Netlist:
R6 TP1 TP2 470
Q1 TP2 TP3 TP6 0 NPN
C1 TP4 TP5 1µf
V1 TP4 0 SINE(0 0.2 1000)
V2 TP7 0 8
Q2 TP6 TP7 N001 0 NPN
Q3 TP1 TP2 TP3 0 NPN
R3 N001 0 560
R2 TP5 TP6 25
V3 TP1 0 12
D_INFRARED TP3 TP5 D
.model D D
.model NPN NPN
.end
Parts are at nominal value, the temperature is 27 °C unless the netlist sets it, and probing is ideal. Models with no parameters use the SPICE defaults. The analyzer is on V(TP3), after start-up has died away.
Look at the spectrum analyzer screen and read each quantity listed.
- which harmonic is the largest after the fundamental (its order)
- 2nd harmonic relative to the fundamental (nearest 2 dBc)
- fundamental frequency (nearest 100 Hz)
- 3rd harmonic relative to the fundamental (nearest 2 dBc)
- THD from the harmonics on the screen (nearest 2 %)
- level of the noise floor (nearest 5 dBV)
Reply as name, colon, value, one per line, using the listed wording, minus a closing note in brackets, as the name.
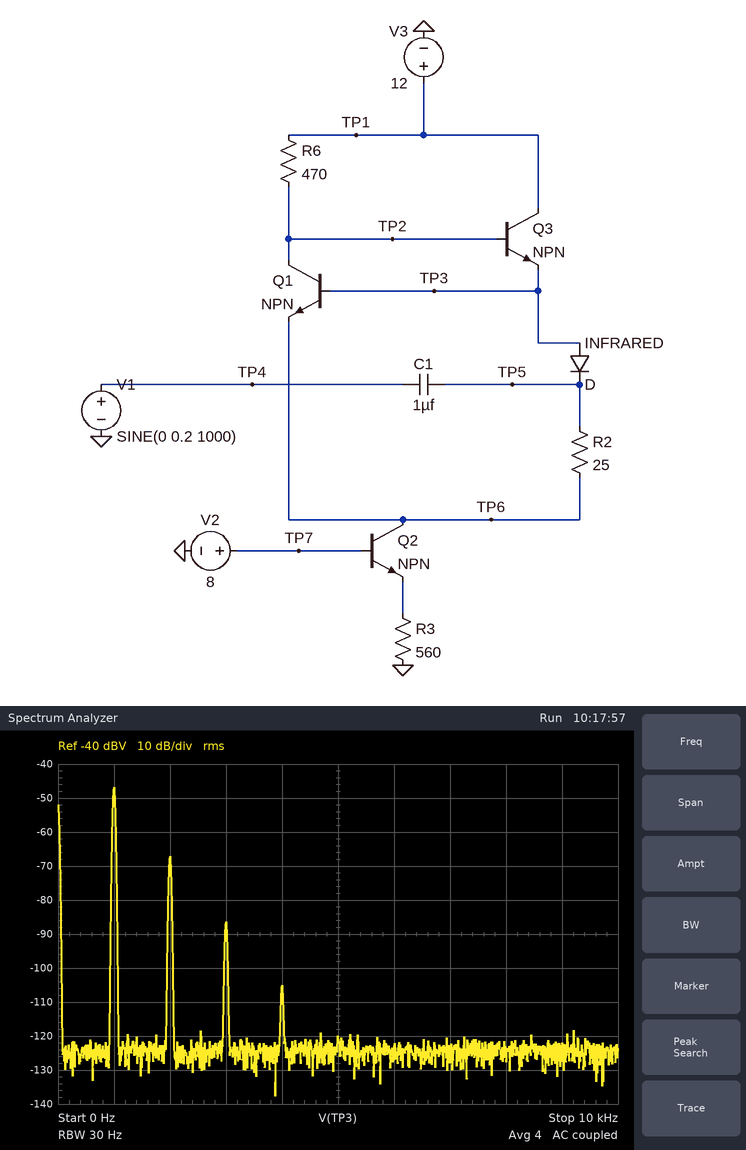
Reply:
which harmonic is the largest after the fundamental: 2
2nd harmonic relative to the fundamental: -20 dBc
fundamental frequency: 1.0 kHz
3rd harmonic relative to the fundamental: -40 dBc
THD from the harmonics on the screen: 10 %
level of the noise floor: -125 dBV
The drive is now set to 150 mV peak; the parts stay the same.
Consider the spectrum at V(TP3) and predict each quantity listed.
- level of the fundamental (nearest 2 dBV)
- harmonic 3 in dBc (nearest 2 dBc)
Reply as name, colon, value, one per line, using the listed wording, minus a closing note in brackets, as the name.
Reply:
level of the fundamental: -50 dBV
harmonic 3 in dBc: -44 dBc
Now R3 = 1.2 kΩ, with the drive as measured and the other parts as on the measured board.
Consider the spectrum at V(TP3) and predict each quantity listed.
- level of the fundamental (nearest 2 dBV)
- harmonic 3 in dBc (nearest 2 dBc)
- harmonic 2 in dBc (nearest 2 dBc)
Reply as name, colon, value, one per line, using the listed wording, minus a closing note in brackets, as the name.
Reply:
level of the fundamental: -24 dBV
harmonic 3 in dBc: -60 dBc
harmonic 2 in dBc: -30 dBc
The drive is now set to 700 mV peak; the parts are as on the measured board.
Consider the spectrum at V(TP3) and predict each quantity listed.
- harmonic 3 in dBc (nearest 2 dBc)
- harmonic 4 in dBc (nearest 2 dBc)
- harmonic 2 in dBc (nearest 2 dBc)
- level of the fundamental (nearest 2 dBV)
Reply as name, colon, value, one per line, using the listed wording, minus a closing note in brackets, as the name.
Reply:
harmonic 3 in dBc: -14 dBc
harmonic 4 in dBc: -22 dBc
harmonic 2 in dBc: -8 dBc
level of the fundamental: -30 dBV
